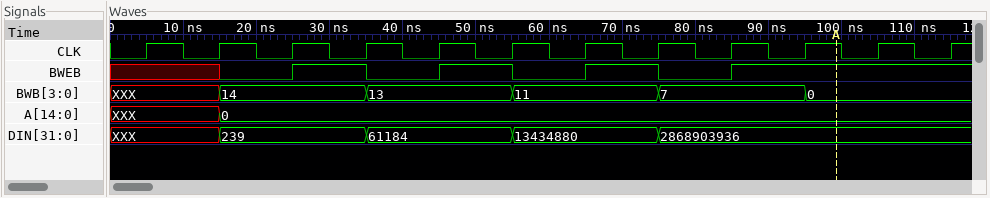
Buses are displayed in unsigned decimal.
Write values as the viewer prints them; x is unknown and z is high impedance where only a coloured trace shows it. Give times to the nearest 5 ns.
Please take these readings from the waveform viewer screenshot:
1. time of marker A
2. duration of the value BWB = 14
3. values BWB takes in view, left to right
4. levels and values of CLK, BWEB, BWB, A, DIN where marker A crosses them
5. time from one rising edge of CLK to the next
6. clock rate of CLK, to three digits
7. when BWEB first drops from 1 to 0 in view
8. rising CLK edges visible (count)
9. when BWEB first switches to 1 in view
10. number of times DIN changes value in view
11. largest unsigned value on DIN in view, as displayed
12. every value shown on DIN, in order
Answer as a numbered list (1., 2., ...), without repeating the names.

1. 100 ns
2. 20 ns
3. XXX, 14, 13, 11, 7, 0
4. CLK=1, BWEB=1, BWB=0, A=0, DIN=2868903936
5. 10 ns
6. 100 MHz
7. 35 ns
8. 12
9. 25 ns
10. 4
11. 2868903936
12. XXX, 239, 61184, 13434880, 2868903936
